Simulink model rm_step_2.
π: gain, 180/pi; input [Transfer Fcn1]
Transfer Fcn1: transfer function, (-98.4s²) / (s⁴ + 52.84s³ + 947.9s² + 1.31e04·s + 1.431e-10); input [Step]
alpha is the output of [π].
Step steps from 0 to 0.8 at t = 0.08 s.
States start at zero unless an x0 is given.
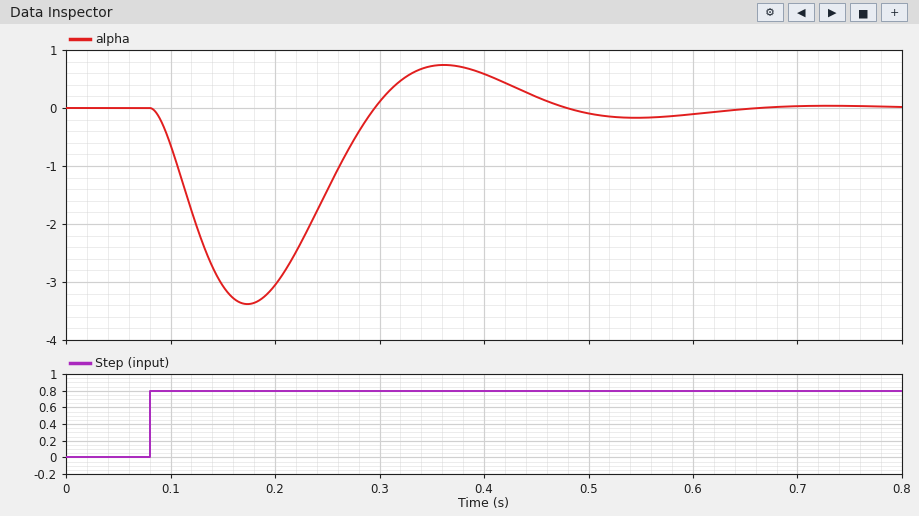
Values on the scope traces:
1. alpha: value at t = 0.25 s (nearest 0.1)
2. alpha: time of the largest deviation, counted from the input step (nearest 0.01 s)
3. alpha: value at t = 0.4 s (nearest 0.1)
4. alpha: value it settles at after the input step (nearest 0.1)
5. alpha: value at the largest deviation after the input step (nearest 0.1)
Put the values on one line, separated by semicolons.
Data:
-1.4; 0.09 s; 0.6; 0.0; -3.4
